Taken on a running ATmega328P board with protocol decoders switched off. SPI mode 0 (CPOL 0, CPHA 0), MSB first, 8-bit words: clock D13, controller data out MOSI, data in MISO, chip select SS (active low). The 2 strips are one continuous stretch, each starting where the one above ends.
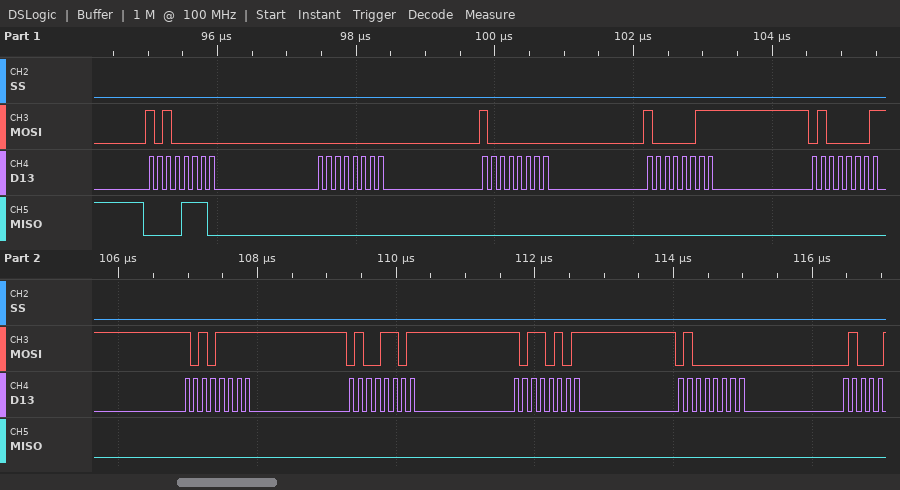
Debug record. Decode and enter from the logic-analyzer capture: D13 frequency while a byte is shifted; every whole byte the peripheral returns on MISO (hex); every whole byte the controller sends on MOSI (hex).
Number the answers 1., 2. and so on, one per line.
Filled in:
1. 8 MHz
2. 0E 00 00 00 00 00 00 00 00
3. A0 00 80 83 41 AF 4D B5 40
